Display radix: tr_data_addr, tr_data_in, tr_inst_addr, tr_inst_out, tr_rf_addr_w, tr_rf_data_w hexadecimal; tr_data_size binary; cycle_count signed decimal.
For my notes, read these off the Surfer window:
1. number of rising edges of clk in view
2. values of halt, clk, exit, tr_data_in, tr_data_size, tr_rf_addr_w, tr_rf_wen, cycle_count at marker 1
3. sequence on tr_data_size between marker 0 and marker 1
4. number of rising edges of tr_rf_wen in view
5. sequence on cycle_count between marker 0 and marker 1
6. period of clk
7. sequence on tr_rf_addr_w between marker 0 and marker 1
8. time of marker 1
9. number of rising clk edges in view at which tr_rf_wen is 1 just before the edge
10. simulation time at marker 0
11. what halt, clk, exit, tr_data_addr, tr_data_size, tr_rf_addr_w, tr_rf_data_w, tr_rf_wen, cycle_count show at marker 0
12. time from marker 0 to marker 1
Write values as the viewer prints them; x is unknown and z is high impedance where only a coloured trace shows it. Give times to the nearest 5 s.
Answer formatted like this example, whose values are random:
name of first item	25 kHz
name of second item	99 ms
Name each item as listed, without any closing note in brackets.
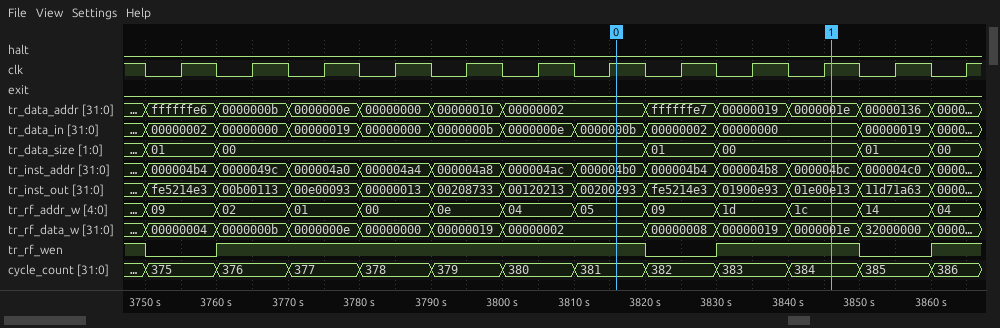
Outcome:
number of rising edges of clk in view	12
values of halt, clk, exit, tr_data_in, tr_data_size, tr_rf_addr_w, tr_rf_wen, cycle_count at marker 1	halt=0, clk=1, exit=0, tr_data_in=00000000, tr_data_size=00, tr_rf_addr_w=1c, tr_rf_wen=1, cycle_count=384
sequence on tr_data_size between marker 0 and marker 1	00, 01, 00
number of rising edges of tr_rf_wen in view	3
sequence on cycle_count between marker 0 and marker 1	381, 382, 383, 384
period of clk	10 s
sequence on tr_rf_addr_w between marker 0 and marker 1	05, 09, 1d, 1c
time of marker 1	3845 s
number of rising clk edges in view at which tr_rf_wen is 1 just before the edge	9
simulation time at marker 0	3815 s
what halt, clk, exit, tr_data_addr, tr_data_size, tr_rf_addr_w, tr_rf_data_w, tr_rf_wen, cycle_count show at marker 0	halt=0, clk=1, exit=0, tr_data_addr=00000002, tr_data_size=00, tr_rf_addr_w=05, tr_rf_data_w=00000002, tr_rf_wen=1, cycle_count=381
time from marker 0 to marker 1	30 s
